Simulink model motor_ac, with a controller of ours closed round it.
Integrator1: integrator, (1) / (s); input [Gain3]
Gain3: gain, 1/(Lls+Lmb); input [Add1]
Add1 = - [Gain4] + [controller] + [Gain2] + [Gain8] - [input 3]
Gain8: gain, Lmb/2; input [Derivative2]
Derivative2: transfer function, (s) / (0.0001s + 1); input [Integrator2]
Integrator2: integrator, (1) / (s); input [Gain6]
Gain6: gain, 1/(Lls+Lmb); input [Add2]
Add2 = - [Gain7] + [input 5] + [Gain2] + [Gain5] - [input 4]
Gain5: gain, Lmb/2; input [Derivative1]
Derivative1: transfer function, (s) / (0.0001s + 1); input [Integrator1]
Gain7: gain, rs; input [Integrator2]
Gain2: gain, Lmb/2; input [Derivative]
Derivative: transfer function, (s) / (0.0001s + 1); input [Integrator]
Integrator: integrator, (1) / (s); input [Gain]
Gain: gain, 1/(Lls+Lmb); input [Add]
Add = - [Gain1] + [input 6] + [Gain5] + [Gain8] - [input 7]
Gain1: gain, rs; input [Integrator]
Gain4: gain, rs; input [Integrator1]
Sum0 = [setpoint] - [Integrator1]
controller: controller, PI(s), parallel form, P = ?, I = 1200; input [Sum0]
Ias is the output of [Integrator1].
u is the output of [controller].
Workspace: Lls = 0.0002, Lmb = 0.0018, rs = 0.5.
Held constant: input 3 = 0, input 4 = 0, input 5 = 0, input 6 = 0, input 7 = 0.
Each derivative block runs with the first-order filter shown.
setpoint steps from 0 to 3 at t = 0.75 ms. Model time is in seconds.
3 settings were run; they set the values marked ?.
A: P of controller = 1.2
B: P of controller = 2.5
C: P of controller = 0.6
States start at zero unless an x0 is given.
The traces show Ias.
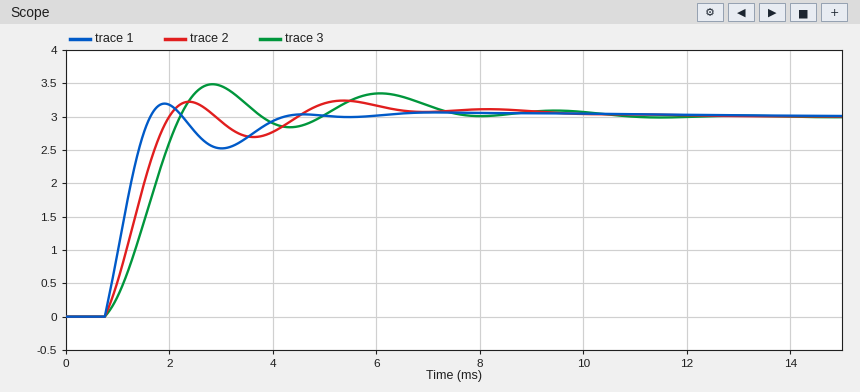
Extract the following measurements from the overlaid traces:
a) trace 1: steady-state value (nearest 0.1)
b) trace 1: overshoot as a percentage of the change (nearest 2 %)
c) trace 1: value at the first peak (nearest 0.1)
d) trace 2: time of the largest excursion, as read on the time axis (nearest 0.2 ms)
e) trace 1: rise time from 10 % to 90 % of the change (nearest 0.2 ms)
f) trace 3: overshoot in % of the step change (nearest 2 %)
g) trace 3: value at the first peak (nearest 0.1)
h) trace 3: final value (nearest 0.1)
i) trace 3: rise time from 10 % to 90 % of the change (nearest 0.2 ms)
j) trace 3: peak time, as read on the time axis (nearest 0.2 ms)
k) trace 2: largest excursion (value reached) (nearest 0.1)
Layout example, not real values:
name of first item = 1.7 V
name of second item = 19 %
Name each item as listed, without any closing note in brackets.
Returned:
trace 1: steady-state value = 3.0
trace 1: overshoot as a percentage of the change = 6 %
trace 1: value at the first peak = 3.2
trace 2: time of the largest excursion, as read on the time axis = 5.4 ms
trace 1: rise time from 10 % to 90 % of the change = 0.6 ms
trace 3: overshoot in % of the step change = 16 %
trace 3: value at the first peak = 3.5
trace 3: final value = 3.0
trace 3: rise time from 10 % to 90 % of the change = 1.0 ms
trace 3: peak time, as read on the time axis = 2.8 ms
trace 2: largest excursion (value reached) = 3.2
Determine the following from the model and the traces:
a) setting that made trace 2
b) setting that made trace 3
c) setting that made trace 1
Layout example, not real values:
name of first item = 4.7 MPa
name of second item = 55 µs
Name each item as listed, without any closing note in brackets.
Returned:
setting that made trace 2 = A
setting that made trace 3 = C
setting that made trace 1 = B
